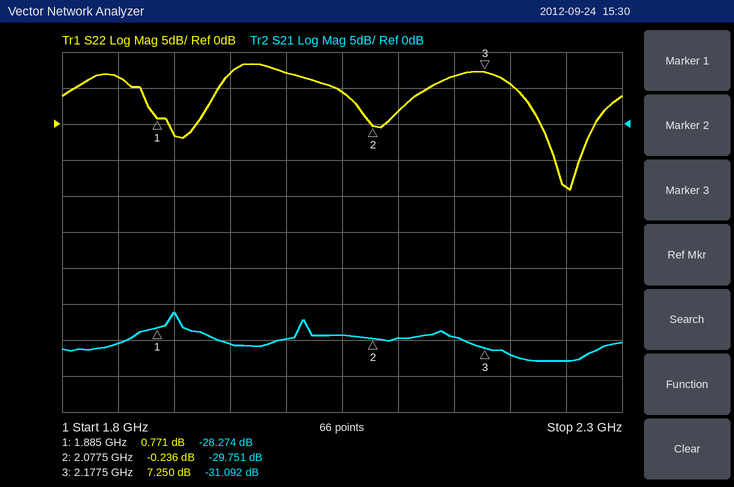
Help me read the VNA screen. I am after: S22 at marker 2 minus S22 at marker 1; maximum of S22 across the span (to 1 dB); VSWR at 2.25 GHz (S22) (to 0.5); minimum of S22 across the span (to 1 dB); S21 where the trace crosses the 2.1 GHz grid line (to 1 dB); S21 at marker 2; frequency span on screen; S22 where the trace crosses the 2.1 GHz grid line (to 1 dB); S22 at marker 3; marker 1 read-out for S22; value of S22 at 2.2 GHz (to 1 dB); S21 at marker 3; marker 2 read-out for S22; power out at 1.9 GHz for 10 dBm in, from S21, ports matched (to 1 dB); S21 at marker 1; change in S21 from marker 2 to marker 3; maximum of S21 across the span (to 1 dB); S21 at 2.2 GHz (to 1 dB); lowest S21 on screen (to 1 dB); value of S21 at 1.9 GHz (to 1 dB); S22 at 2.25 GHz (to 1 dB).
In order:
-1.007 dB
8 dB
2.0
-9 dB
-30 dB
-29.751 dB
500 MHz
2 dB
7.250 dB
0.771 dB
6 dB
-31.092 dB
-0.236 dB
-16 dBm
-28.274 dB
-1.341 dB
-26 dB
-32 dB
-33 dB
-26 dB
-9 dB
